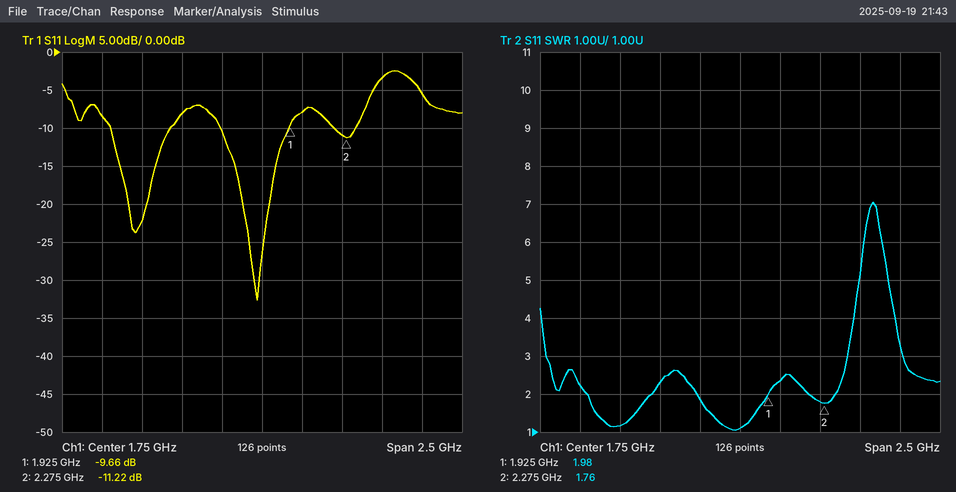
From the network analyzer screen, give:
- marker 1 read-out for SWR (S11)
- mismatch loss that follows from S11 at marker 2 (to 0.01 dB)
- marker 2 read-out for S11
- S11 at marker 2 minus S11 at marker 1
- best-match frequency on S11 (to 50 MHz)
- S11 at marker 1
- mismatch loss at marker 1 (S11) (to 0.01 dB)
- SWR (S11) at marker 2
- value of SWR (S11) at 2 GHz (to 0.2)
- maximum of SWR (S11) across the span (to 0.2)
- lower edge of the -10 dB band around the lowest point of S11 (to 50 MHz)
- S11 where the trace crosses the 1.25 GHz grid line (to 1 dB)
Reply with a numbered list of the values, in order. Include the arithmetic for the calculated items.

1. 1.98
2. −10 log10(1 − 10^(-11.22/10)) ≈ 0.34 dB
3. -11.22 dB
4. -11.22 − (-9.66) = -1.56 dB
5. 1.70 GHz
6. -9.66 dB
7. −10 log10(1 − 10^(-9.66/10)) ≈ 0.50 dB
8. 1.76
9. 2.4
10. 7.0
11. 1.50 GHz
12. -8 dB
